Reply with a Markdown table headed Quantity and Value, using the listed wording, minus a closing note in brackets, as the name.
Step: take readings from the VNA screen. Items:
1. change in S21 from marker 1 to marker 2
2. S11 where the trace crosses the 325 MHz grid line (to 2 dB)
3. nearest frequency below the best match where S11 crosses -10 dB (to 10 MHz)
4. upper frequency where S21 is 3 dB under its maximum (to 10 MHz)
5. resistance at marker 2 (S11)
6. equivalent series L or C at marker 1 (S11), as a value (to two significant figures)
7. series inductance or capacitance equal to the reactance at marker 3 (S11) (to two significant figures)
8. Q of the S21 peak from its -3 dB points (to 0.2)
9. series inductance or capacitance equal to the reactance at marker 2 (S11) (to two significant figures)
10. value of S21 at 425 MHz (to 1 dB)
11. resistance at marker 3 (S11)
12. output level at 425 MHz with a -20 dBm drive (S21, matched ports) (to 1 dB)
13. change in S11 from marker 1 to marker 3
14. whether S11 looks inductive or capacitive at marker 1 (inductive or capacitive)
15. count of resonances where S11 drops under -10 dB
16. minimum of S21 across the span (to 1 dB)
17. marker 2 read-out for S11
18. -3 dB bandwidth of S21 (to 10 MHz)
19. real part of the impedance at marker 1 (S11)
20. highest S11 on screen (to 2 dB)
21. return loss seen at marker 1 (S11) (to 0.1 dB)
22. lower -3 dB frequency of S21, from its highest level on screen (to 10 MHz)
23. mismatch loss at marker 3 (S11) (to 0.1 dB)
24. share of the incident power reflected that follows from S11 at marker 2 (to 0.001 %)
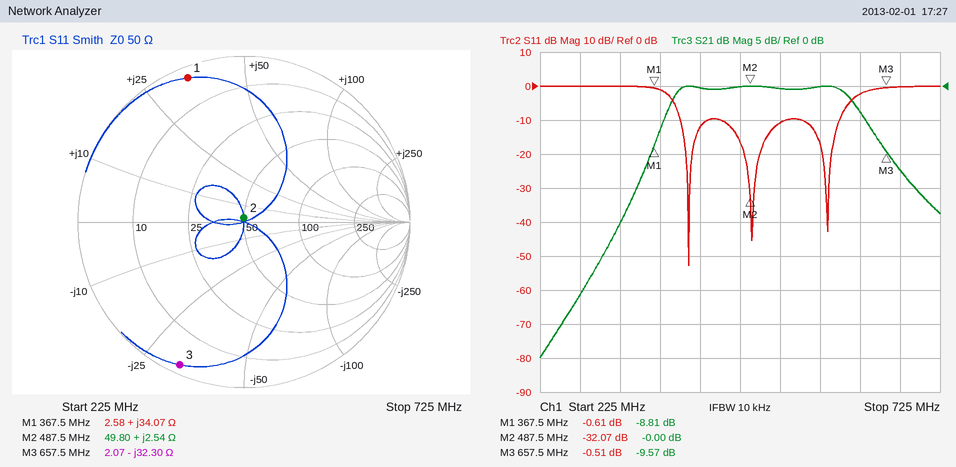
| Quantity | Value |
|---|---|
| change in S21 from marker 1 to marker 2 | 8.81 dB |
| S11 where the trace crosses the 325 MHz grid line | 0 dB |
| nearest frequency below the best match where S11 crosses -10 dB | 400 MHz |
| upper frequency where S21 is 3 dB under its maximum | 620 MHz |
| resistance at marker 2 | 49.80 Ω |
| equivalent series L or C at marker 1 (S11), as a value | 15 nH |
| series inductance or capacitance equal to the reactance at marker 3 (S11) | 7.5 pF |
| Q of the S21 peak from its -3 dB points | 2.2 |
| series inductance or capacitance equal to the reactance at marker 2 (S11) | 830 pH |
| value of S21 at 425 MHz | 0 dB |
| resistance at marker 3 | 2.07 Ω |
| output level at 425 MHz with a -20 dBm drive (S21, matched ports) | -20 dBm |
| change in S11 from marker 1 to marker 3 | 0.10 dB |
| whether S11 looks inductive or capacitive at marker 1 | inductive |
| count of resonances where S11 drops under -10 dB | 3 |
| minimum of S21 across the span | -40 dB |
| marker 2 read-out for S11 | -32.07 dB |
| -3 dB bandwidth of S21 | 230 MHz |
| real part of the impedance at marker 1 | 2.58 Ω |
| highest S11 on screen | 0 dB |
| return loss seen at marker 1 (S11) | 0.6 dB |
| lower -3 dB frequency of S21, from its highest level on screen | 390 MHz |
| mismatch loss at marker 3 (S11) | 9.6 dB |
| share of the incident power reflected that follows from S11 at marker 2 | 0.062 % |
